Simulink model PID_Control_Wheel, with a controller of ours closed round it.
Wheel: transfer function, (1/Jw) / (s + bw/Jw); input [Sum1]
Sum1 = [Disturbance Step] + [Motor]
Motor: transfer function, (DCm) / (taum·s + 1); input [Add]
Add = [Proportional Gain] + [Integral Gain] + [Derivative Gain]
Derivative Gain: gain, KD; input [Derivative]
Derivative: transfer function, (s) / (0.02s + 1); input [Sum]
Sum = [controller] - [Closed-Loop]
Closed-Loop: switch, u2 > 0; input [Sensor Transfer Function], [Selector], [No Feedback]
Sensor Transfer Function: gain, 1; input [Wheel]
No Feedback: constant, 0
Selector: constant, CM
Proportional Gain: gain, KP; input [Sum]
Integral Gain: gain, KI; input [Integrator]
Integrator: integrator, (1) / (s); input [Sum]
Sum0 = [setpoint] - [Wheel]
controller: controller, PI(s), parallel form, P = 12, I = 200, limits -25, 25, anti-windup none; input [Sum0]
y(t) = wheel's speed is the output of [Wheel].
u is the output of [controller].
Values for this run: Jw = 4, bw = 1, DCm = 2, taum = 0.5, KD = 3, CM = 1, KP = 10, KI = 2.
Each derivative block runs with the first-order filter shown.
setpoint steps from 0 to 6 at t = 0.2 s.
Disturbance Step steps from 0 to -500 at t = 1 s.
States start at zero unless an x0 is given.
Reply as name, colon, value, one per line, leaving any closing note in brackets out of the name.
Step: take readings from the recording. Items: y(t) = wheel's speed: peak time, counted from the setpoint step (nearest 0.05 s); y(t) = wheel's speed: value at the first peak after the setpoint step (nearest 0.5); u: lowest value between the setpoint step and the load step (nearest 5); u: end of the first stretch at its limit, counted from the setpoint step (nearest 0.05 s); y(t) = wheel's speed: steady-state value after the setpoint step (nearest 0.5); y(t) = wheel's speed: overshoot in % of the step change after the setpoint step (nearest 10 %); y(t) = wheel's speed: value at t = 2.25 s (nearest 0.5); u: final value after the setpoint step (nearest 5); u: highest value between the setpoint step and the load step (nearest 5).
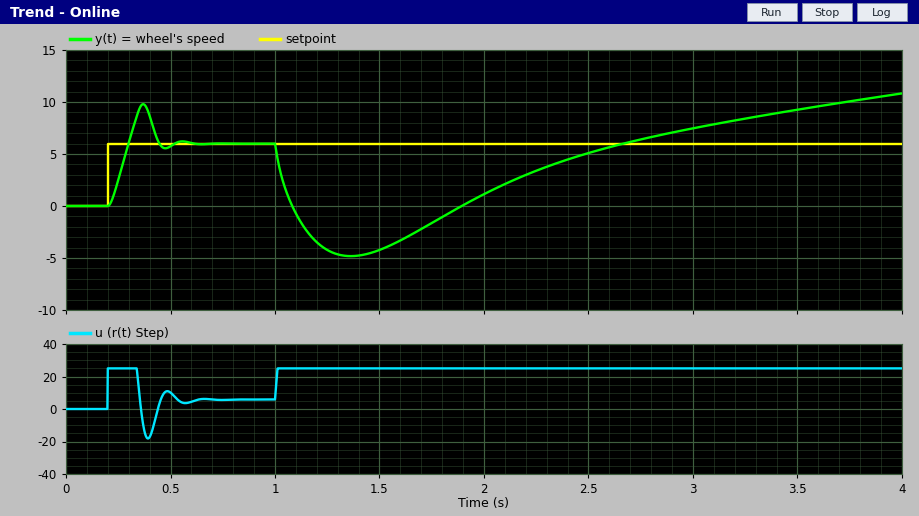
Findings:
y(t) = wheel's speed: peak time, counted from the setpoint step: 0.15 s
y(t) = wheel's speed: value at the first peak after the setpoint step: 10.0
u: lowest value between the setpoint step and the load step: -20
u: end of the first stretch at its limit, counted from the setpoint step: 0.15 s
y(t) = wheel's speed: steady-state value after the setpoint step: 6.0
y(t) = wheel's speed: overshoot in % of the step change after the setpoint step: 60 %
y(t) = wheel's speed: value at t = 2.25 s: 3.5
u: final value after the setpoint step: 5
u: highest value between the setpoint step and the load step: 25
